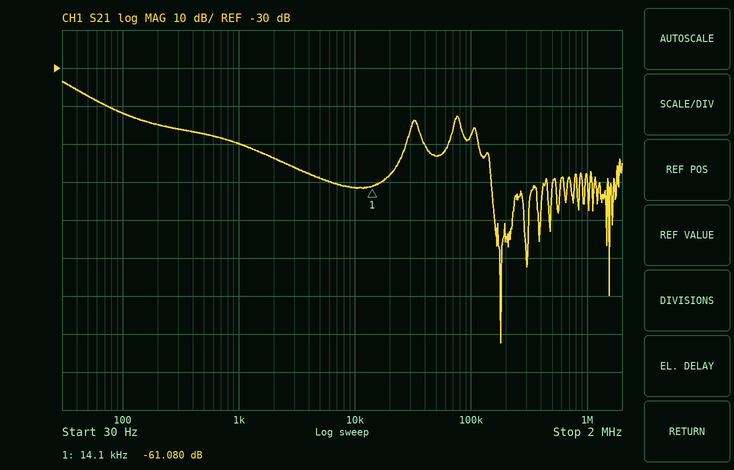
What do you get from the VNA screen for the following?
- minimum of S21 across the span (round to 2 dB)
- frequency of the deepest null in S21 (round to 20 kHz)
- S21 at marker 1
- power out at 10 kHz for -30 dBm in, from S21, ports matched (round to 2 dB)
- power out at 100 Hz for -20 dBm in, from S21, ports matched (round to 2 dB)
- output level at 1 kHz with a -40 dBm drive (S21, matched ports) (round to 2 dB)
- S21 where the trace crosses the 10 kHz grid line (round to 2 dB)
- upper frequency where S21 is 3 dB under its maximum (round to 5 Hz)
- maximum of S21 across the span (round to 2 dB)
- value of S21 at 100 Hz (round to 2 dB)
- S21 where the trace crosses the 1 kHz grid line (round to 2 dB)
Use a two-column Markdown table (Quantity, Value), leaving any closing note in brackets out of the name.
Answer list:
| Quantity | Value |
|---|---|
| minimum of S21 across the span | -102 dB |
| frequency of the deepest null in S21 | 180 kHz |
| S21 at marker 1 | -61.080 dB |
| power out at 10 kHz for -30 dBm in, from S21, ports matched | -92 dBm |
| power out at 100 Hz for -20 dBm in, from S21, ports matched | -62 dBm |
| output level at 1 kHz with a -40 dBm drive (S21, matched ports) | -90 dBm |
| S21 where the trace crosses the 10 kHz grid line | -62 dB |
| upper frequency where S21 is 3 dB under its maximum | 45 Hz |
| maximum of S21 across the span | -34 dB |
| value of S21 at 100 Hz | -42 dB |
| S21 where the trace crosses the 1 kHz grid line | -50 dB |
